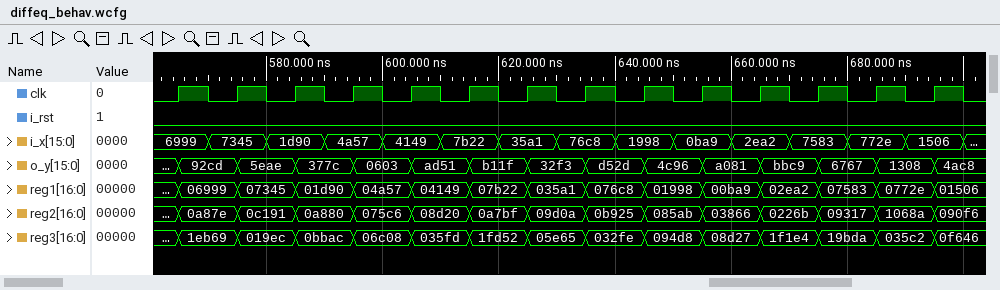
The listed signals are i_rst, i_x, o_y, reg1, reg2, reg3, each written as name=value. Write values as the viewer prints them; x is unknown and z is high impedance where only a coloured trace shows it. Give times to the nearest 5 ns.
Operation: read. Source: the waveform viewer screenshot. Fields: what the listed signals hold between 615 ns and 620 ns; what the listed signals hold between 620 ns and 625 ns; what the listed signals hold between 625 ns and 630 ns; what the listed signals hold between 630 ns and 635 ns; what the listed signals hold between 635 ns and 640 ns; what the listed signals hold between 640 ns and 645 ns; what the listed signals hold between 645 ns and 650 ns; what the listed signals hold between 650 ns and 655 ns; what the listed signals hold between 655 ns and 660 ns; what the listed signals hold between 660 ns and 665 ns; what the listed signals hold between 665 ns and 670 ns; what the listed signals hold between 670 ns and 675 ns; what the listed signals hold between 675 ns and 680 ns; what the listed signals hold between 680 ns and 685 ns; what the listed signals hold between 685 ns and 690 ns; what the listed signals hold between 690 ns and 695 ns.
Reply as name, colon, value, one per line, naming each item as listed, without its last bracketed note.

what the listed signals hold between 615 ns and 620 ns: i_rst=0, i_x=7b22, o_y=b11f, reg1=07b22, reg2=0a7bf, reg3=1fd52
what the listed signals hold between 620 ns and 625 ns: i_rst=0, i_x=35a1, o_y=b11f, reg1=07b22, reg2=0a7bf, reg3=1fd52
what the listed signals hold between 625 ns and 630 ns: i_rst=0, i_x=35a1, o_y=32f3, reg1=035a1, reg2=09d0a, reg3=05e65
what the listed signals hold between 630 ns and 635 ns: i_rst=0, i_x=76c8, o_y=32f3, reg1=035a1, reg2=09d0a, reg3=05e65
what the listed signals hold between 635 ns and 640 ns: i_rst=0, i_x=76c8, o_y=d52d, reg1=076c8, reg2=0b925, reg3=032fe
what the listed signals hold between 640 ns and 645 ns: i_rst=0, i_x=1998, o_y=d52d, reg1=076c8, reg2=0b925, reg3=032fe
what the listed signals hold between 645 ns and 650 ns: i_rst=0, i_x=1998, o_y=4c96, reg1=01998, reg2=085ab, reg3=094d8
what the listed signals hold between 650 ns and 655 ns: i_rst=0, i_x=0ba9, o_y=4c96, reg1=01998, reg2=085ab, reg3=094d8
what the listed signals hold between 655 ns and 660 ns: i_rst=0, i_x=0ba9, o_y=a081, reg1=00ba9, reg2=03866, reg3=08d27
what the listed signals hold between 660 ns and 665 ns: i_rst=0, i_x=2ea2, o_y=a081, reg1=00ba9, reg2=03866, reg3=08d27
what the listed signals hold between 665 ns and 670 ns: i_rst=0, i_x=2ea2, o_y=bbc9, reg1=02ea2, reg2=0226b, reg3=1f1e4
what the listed signals hold between 670 ns and 675 ns: i_rst=0, i_x=7583, o_y=bbc9, reg1=02ea2, reg2=0226b, reg3=1f1e4
what the listed signals hold between 675 ns and 680 ns: i_rst=0, i_x=7583, o_y=6767, reg1=07583, reg2=09317, reg3=19bda
what the listed signals hold between 680 ns and 685 ns: i_rst=0, i_x=772e, o_y=6767, reg1=07583, reg2=09317, reg3=19bda
what the listed signals hold between 685 ns and 690 ns: i_rst=0, i_x=772e, o_y=1308, reg1=0772e, reg2=1068a, reg3=035c2
what the listed signals hold between 690 ns and 695 ns: i_rst=0, i_x=1506, o_y=1308, reg1=0772e, reg2=1068a, reg3=035c2
